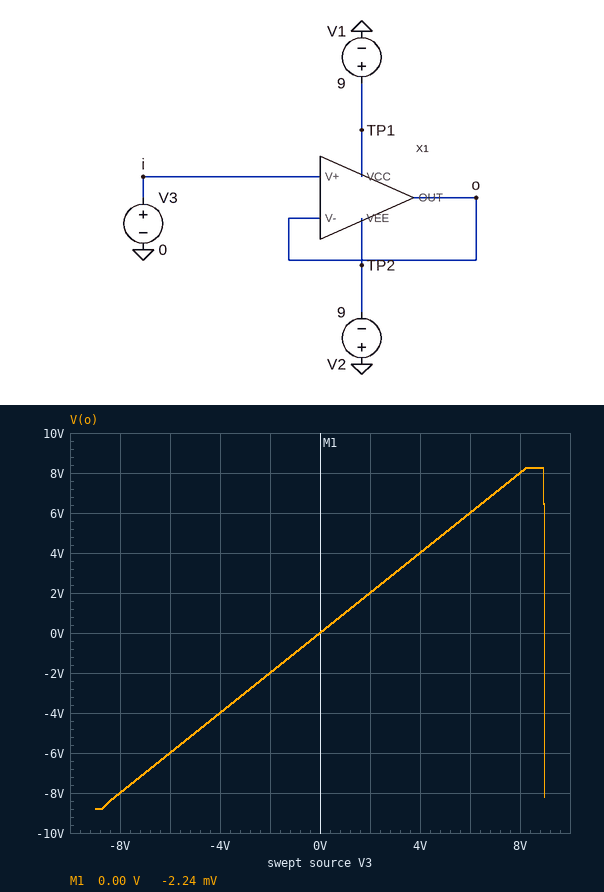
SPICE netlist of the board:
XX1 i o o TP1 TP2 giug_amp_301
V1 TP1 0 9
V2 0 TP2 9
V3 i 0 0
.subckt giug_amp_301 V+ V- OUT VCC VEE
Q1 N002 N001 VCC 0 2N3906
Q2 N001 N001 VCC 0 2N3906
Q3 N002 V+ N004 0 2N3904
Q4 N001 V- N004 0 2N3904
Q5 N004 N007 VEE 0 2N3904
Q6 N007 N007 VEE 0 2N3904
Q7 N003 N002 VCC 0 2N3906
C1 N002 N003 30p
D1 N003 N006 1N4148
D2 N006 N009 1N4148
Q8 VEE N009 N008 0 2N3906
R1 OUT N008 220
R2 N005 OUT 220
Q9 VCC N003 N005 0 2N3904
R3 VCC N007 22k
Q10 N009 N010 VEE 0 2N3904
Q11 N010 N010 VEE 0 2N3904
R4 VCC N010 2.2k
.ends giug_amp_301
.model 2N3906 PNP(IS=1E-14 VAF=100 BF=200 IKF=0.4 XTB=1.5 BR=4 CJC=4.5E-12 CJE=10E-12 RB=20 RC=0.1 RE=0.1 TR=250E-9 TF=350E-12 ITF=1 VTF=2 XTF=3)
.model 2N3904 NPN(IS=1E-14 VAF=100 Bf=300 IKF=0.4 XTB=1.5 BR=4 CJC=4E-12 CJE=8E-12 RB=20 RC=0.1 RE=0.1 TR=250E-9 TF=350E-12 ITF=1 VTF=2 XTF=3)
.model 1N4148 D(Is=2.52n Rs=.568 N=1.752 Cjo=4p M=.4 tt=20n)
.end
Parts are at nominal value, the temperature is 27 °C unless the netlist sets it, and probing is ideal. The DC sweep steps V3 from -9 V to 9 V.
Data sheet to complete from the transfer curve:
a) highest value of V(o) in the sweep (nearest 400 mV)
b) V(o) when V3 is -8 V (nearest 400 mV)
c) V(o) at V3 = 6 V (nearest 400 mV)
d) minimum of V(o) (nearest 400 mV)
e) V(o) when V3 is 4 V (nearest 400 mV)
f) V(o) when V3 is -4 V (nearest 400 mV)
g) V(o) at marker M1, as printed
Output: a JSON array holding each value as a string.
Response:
["8.4 V", "-8.0 V", "6.0 V", "-8.8 V", "4.0 V", "-4.0 V", "-2.24 mV"]
